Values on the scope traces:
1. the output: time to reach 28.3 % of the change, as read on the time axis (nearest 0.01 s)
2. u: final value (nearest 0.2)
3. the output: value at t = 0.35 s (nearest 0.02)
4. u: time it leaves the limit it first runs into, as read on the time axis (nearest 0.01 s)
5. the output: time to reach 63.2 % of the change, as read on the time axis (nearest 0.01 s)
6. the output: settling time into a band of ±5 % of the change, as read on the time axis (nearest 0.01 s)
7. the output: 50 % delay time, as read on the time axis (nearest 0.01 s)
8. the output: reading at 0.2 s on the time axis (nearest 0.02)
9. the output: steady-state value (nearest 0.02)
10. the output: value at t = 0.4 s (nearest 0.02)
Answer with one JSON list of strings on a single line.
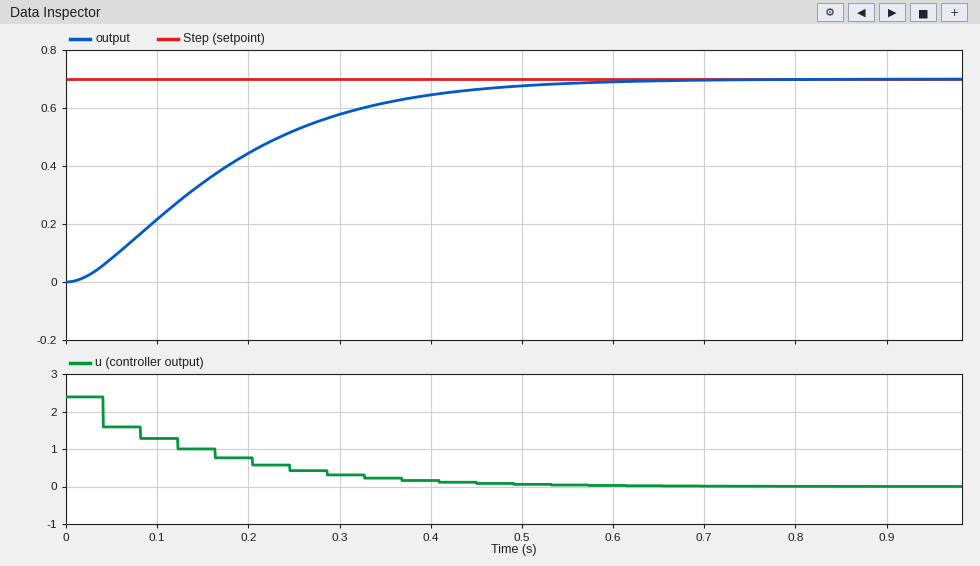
["0.09 s", "0.0", "0.62", "0.04 s", "0.20 s", "0.45 s", "0.15 s", "0.44", "0.70", "0.64"]
